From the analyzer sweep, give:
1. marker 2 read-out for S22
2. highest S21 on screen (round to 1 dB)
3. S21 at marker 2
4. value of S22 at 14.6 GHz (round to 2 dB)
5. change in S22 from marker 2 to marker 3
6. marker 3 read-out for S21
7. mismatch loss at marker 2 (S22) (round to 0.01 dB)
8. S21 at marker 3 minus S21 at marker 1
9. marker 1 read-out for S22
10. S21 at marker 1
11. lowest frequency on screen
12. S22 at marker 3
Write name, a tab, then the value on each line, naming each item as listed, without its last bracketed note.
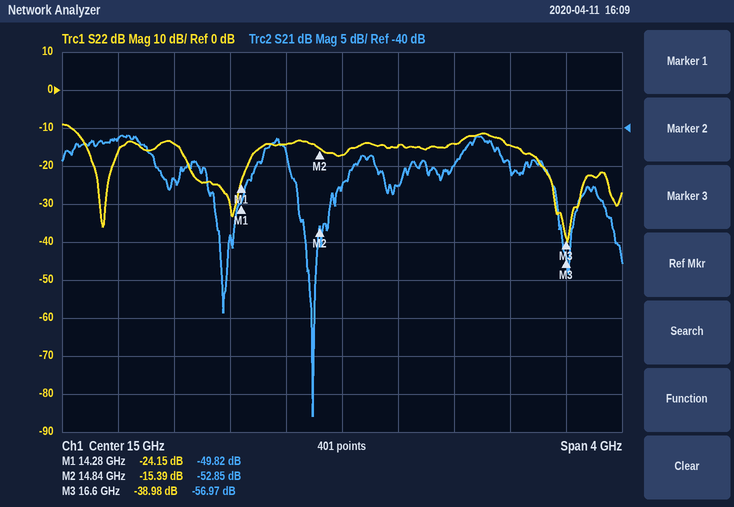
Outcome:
marker 2 read-out for S22	-15.39 dB
highest S21 on screen	-41 dB
S21 at marker 2	-52.85 dB
value of S22 at 14.6 GHz	-14 dB
change in S22 from marker 2 to marker 3	-23.59 dB
marker 3 read-out for S21	-56.97 dB
mismatch loss at marker 2 (S22)	0.13 dB
S21 at marker 3 minus S21 at marker 1	-7.15 dB
marker 1 read-out for S22	-24.15 dB
S21 at marker 1	-49.82 dB
lowest frequency on screen	13 GHz
S22 at marker 3	-38.98 dB
